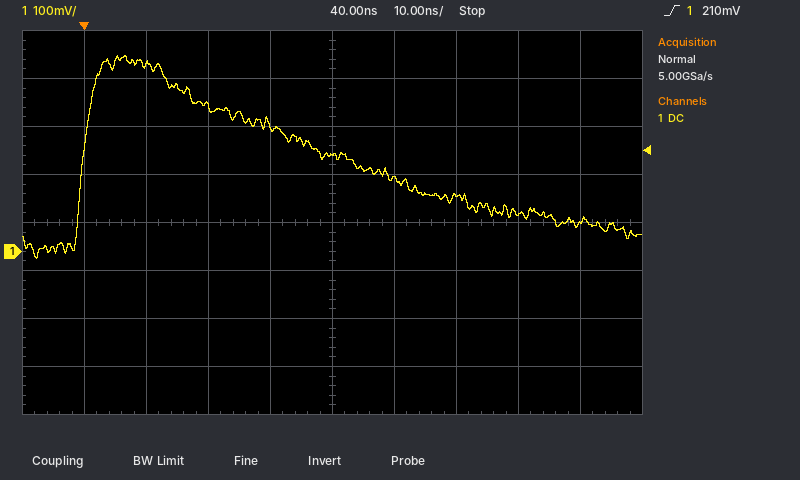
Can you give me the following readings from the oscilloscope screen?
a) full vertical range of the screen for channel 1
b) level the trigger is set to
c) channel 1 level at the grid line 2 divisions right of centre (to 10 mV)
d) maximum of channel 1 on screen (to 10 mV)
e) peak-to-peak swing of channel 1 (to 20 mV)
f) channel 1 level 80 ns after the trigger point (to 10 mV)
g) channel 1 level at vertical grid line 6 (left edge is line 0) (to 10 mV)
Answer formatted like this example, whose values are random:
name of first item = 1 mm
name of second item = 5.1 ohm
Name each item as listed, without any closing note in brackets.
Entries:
full vertical range of the screen for channel 1 = 800 mV
level the trigger is set to = 210 mV
channel 1 level at the grid line 2 divisions right of centre = 120 mV
maximum of channel 1 on screen = 410 mV
peak-to-peak swing of channel 1 = 420 mV
channel 1 level 80 ns after the trigger point = 60 mV
channel 1 level at vertical grid line 6 (left edge is line 0) = 150 mV
